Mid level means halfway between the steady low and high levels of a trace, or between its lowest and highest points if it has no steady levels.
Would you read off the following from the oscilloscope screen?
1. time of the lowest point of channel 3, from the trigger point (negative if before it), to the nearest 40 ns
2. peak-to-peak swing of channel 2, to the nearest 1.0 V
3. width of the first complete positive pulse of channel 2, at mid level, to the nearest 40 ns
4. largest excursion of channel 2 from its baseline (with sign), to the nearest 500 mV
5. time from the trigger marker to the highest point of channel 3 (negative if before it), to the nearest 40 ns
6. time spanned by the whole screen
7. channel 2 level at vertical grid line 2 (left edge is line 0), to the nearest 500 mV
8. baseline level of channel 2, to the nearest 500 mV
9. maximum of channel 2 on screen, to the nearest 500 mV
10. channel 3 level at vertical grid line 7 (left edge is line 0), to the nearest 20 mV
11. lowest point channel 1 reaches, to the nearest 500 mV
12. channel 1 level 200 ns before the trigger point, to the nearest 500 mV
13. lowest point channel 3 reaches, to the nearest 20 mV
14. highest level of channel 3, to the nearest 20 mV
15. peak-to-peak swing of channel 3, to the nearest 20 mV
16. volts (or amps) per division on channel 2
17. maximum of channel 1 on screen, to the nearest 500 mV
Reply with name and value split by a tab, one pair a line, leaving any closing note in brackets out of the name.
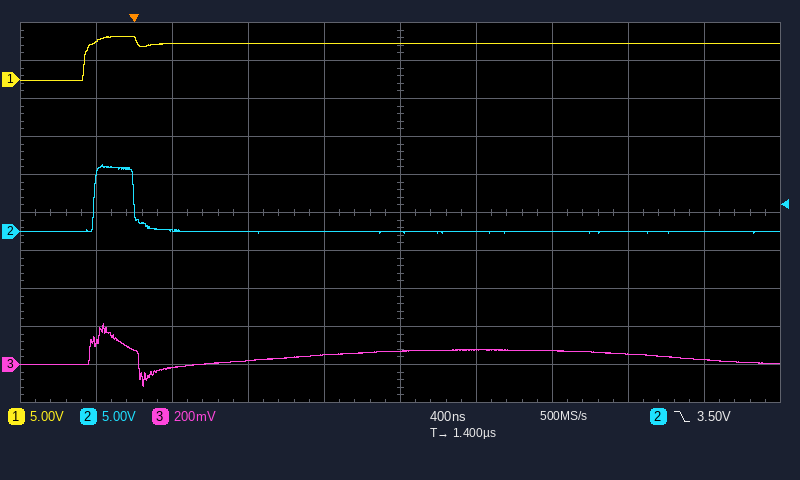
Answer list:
time of the lowest point of channel 3, from the trigger point (negative if before it), to the nearest 40 ns	+40 ns
peak-to-peak swing of channel 2, to the nearest 1.0 V	9.0 V
width of the first complete positive pulse of channel 2, at mid level, to the nearest 40 ns	200 ns
largest excursion of channel 2 from its baseline (with sign), to the nearest 500 mV	+9.0 V
time from the trigger marker to the highest point of channel 3 (negative if before it), to the nearest 40 ns	-160 ns
time spanned by the whole screen	4 µs
channel 2 level at vertical grid line 2 (left edge is line 0), to the nearest 500 mV	0.0 V
baseline level of channel 2, to the nearest 500 mV	0.0 V
maximum of channel 2 on screen, to the nearest 500 mV	9.0 V
channel 3 level at vertical grid line 7 (left edge is line 0), to the nearest 20 mV	80 mV
lowest point channel 1 reaches, to the nearest 500 mV	0.0 V
channel 1 level 200 ns before the trigger point, to the nearest 500 mV	5.0 V
lowest point channel 3 reaches, to the nearest 20 mV	-120 mV
highest level of channel 3, to the nearest 20 mV	220 mV
peak-to-peak swing of channel 3, to the nearest 20 mV	340 mV
volts (or amps) per division on channel 2	5 V
maximum of channel 1 on screen, to the nearest 500 mV	5.5 V
